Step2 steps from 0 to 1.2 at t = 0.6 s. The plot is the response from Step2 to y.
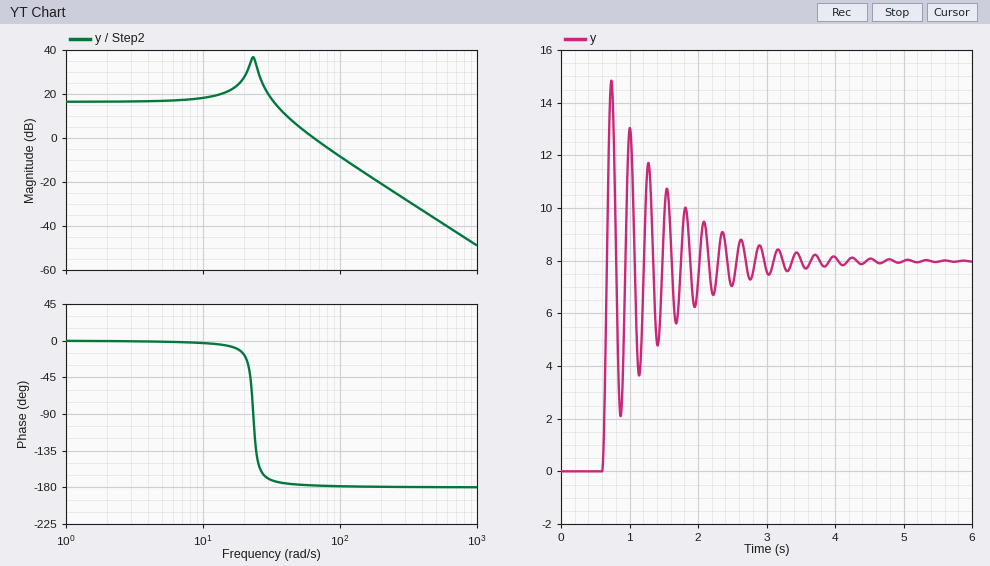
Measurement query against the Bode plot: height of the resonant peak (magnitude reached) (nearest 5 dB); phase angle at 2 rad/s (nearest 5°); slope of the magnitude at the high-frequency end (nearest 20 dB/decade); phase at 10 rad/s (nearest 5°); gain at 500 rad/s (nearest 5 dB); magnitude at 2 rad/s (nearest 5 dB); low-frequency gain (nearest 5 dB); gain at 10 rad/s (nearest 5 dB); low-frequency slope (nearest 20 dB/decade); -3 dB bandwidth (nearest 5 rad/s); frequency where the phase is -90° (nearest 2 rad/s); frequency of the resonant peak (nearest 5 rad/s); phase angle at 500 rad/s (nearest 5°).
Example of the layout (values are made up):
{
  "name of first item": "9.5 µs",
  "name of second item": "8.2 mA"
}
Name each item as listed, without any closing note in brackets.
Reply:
{
  "height of the resonant peak (magnitude reached)": "35 dB",
  "phase angle at 2 rad/s": "0°",
  "slope of the magnitude at the high-frequency end": "-40 dB/decade",
  "phase at 10 rad/s": "-5°",
  "gain at 500 rad/s": "-35 dB",
  "magnitude at 2 rad/s": "15 dB",
  "low-frequency gain": "15 dB",
  "gain at 10 rad/s": "20 dB",
  "low-frequency slope": "0 dB/decade",
  "-3 dB bandwidth": "35 rad/s",
  "frequency where the phase is -90°": "24 rad/s",
  "frequency of the resonant peak": "25 rad/s",
  "phase angle at 500 rad/s": "-180°"
}
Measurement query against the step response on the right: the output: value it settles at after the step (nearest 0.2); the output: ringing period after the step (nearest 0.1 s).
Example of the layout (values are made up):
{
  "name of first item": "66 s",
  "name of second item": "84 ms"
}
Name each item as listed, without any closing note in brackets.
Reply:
{
  "the output: value it settles at after the step": "8.0",
  "the output: ringing period after the step": "0.3 s"
}
